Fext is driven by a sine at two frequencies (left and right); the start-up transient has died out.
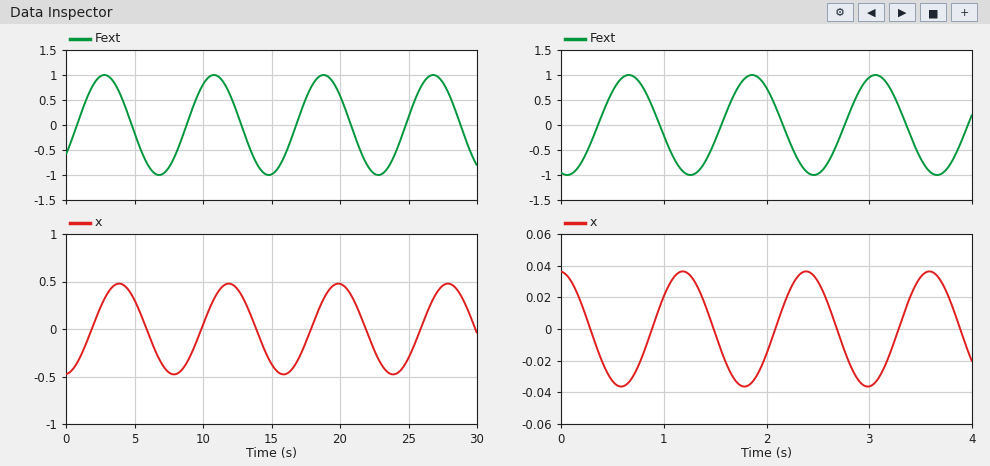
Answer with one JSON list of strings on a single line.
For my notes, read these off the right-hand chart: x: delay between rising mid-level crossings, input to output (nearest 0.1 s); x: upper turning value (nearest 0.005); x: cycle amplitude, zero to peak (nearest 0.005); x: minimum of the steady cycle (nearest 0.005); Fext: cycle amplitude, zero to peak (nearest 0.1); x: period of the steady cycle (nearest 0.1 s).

["0.5 s", "0.035", "0.035", "-0.035", "1.0", "1.2 s"]
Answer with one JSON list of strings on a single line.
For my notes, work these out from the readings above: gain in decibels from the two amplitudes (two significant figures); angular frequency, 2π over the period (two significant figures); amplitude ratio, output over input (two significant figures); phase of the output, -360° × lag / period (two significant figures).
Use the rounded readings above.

["-29 dB", "5.2 rad/s", "0.035", "-150°"]
